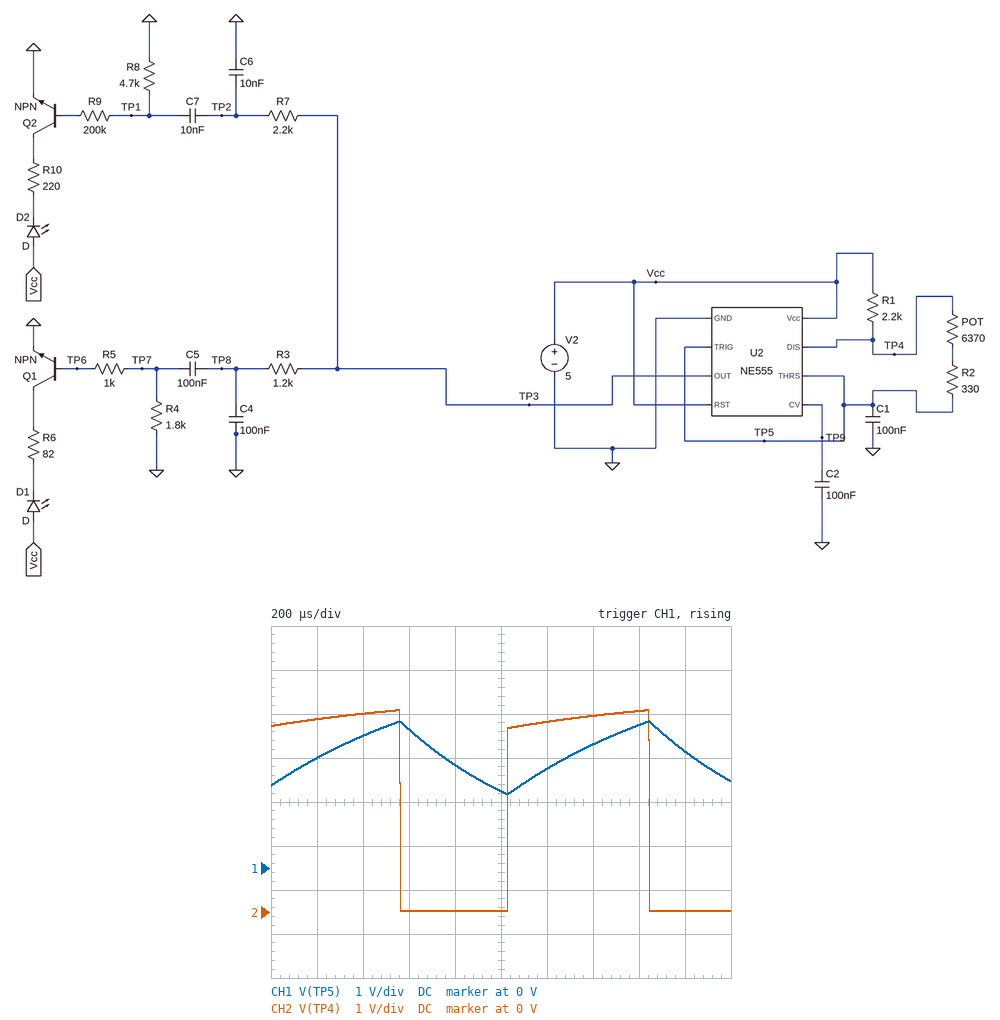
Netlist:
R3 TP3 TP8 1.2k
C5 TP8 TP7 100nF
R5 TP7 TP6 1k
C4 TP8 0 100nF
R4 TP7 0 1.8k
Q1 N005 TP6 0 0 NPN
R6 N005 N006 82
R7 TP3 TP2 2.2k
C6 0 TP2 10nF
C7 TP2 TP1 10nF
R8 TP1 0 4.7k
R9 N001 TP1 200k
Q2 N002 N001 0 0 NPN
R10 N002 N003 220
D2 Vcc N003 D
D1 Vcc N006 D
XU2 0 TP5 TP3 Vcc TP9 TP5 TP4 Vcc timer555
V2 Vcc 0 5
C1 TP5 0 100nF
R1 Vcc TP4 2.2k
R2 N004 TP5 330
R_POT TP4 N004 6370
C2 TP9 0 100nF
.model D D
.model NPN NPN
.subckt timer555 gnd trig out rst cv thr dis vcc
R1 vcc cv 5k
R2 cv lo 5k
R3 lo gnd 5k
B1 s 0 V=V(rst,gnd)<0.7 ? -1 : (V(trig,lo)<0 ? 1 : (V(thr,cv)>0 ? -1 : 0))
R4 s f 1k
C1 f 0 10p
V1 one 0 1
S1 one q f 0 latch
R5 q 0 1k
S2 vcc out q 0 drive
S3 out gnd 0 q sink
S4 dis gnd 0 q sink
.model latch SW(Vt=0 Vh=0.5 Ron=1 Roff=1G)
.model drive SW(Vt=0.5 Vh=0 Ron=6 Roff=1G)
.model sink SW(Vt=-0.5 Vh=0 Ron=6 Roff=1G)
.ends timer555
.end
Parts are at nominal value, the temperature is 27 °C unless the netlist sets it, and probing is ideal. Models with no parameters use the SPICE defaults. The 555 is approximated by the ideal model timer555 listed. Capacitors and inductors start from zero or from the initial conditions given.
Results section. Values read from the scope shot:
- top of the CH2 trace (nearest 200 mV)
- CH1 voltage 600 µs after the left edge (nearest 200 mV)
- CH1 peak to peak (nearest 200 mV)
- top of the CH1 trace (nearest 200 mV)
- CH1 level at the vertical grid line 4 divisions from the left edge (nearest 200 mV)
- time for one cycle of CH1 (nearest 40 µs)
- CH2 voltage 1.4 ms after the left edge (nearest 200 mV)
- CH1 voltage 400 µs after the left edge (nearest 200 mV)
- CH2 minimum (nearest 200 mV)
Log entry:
4.6 V
3.2 V
1.6 V
3.4 V
2.4 V
1.08 ms
4.4 V
3.0 V
0 V
